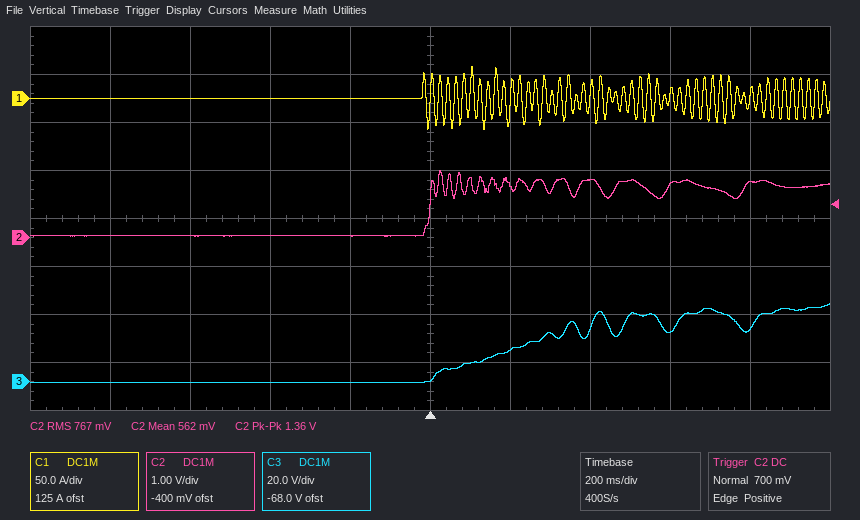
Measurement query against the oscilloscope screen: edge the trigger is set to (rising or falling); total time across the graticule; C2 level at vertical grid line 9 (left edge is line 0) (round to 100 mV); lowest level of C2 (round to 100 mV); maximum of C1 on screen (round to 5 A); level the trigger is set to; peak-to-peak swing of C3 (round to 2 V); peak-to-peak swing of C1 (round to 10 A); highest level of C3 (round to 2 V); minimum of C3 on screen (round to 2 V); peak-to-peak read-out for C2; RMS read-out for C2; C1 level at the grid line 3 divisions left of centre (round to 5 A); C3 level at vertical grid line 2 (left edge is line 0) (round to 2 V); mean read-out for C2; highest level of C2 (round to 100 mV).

rising
2 s
1.1 V
0.0 V
35 A
700 mV
32 V
70 A
32 V
0 V
1.36 V
767 mV
0 A
0 V
562 mV
1.4 V
